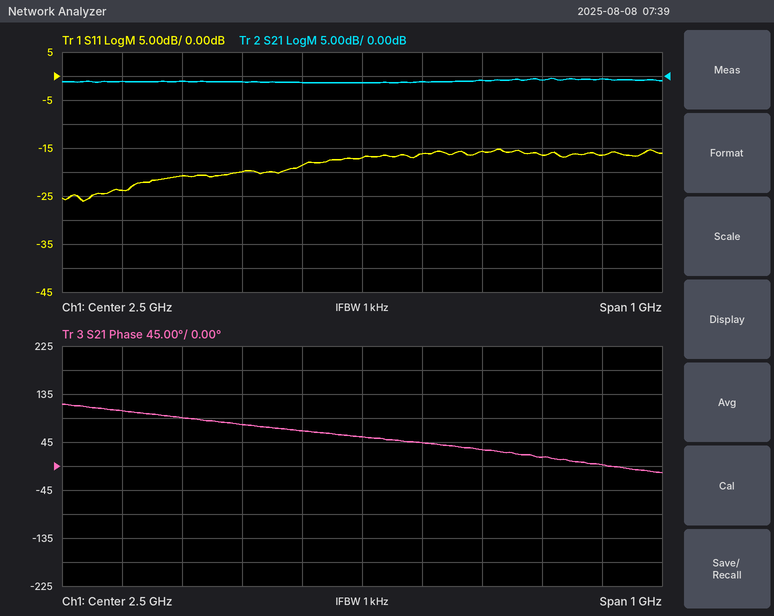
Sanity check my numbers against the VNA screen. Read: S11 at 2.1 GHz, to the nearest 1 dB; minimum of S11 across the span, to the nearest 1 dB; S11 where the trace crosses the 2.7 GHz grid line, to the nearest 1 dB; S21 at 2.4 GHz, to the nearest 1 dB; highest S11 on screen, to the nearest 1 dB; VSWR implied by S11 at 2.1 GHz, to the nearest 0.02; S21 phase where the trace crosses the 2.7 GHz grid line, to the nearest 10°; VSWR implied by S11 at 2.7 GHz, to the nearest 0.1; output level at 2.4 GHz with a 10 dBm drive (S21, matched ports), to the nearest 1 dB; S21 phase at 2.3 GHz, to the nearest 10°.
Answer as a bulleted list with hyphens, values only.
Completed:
- -24 dB
- -26 dB
- -16 dB
- -1 dB
- -15 dB
- 1.14
- 30°
- 1.4
- 9 dBm
- 80°
